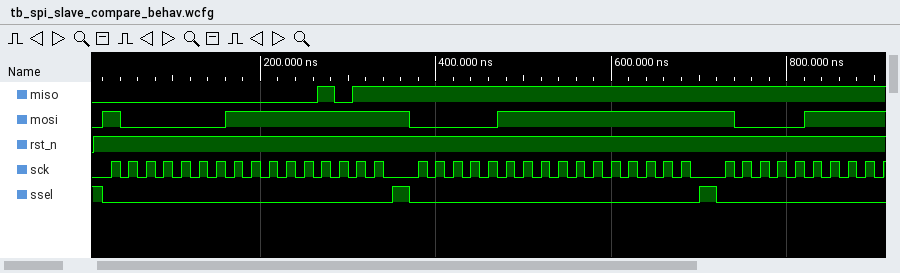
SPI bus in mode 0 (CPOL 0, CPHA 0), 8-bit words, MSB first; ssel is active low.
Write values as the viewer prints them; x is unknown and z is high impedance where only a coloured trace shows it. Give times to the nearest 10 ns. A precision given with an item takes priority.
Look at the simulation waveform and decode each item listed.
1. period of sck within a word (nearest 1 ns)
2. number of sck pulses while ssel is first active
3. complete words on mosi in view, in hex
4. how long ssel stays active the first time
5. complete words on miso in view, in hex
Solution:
20 ns
16
81, FF, 07, FF, 87
330 ns
00, 0B, FF, FF, FF
